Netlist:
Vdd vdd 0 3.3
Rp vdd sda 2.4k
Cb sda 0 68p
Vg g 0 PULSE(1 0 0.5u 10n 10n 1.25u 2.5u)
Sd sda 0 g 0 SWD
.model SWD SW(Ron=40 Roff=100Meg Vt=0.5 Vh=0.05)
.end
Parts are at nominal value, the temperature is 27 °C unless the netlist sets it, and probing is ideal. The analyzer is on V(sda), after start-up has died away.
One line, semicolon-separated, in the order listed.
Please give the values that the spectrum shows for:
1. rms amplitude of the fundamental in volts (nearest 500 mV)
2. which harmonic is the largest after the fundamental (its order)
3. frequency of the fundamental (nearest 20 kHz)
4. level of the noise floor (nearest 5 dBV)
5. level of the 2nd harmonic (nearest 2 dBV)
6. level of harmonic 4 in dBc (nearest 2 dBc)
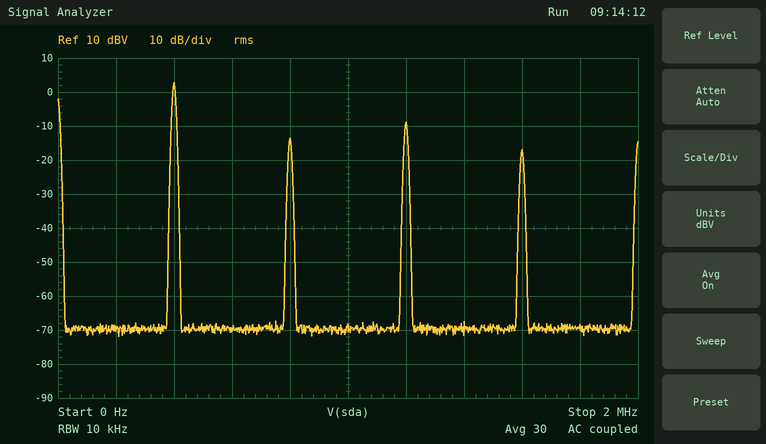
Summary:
1.5 V; 3; 400 kHz; -70 dBV; -14 dBV; -20 dBc
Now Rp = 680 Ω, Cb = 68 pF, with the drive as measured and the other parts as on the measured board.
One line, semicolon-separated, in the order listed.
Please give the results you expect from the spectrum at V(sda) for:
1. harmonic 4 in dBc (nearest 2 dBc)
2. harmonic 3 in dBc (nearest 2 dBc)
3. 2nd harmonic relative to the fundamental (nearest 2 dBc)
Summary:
-28 dBc; -10 dBc; -28 dBc
